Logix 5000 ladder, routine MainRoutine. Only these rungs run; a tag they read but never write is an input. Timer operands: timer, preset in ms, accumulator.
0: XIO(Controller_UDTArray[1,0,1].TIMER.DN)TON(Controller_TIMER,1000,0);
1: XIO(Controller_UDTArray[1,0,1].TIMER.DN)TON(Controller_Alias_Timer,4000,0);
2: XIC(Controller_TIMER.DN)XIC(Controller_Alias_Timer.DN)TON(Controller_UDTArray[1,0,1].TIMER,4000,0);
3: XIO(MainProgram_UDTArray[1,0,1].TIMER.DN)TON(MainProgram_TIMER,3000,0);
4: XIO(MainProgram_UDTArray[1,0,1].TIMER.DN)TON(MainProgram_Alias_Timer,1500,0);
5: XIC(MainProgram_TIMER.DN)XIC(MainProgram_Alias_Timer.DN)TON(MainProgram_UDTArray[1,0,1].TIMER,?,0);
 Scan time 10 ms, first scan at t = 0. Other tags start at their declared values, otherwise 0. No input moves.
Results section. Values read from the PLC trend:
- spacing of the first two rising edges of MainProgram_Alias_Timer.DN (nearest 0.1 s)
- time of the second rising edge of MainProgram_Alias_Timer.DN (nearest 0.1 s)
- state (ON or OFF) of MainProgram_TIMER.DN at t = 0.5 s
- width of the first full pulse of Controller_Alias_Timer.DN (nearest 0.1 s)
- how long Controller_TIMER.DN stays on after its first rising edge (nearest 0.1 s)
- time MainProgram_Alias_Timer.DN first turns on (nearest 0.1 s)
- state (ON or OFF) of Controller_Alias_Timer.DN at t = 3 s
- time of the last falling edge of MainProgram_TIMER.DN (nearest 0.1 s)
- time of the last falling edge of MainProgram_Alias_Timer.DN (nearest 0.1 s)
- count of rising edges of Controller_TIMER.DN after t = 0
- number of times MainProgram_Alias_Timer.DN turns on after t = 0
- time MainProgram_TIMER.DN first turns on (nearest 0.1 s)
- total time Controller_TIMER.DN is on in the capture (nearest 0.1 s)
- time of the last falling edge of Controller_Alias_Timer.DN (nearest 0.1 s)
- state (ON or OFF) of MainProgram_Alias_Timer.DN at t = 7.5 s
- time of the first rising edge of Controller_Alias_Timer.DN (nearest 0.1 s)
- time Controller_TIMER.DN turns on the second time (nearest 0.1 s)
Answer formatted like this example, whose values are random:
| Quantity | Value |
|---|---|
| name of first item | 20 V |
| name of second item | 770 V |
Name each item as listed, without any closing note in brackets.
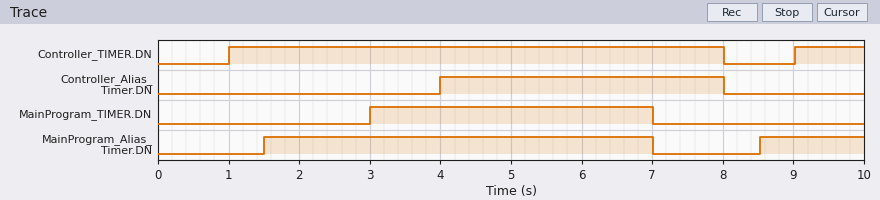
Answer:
| Quantity | Value |
|---|---|
| spacing of the first two rising edges of MainProgram_Alias_Timer.DN | 7.0 s |
| time of the second rising edge of MainProgram_Alias_Timer.DN | 8.5 s |
| state (ON or OFF) of MainProgram_TIMER.DN at t = 0.5 s | OFF |
| width of the first full pulse of Controller_Alias_Timer.DN | 4.0 s |
| how long Controller_TIMER.DN stays on after its first rising edge | 7.0 s |
| time MainProgram_Alias_Timer.DN first turns on | 1.5 s |
| state (ON or OFF) of Controller_Alias_Timer.DN at t = 3 s | OFF |
| time of the last falling edge of MainProgram_TIMER.DN | 7.0 s |
| time of the last falling edge of MainProgram_Alias_Timer.DN | 7.0 s |
| count of rising edges of Controller_TIMER.DN after t = 0 | 2 |
| number of times MainProgram_Alias_Timer.DN turns on after t = 0 | 2 |
| time MainProgram_TIMER.DN first turns on | 3.0 s |
| total time Controller_TIMER.DN is on in the capture | 8.0 s |
| time of the last falling edge of Controller_Alias_Timer.DN | 8.0 s |
| state (ON or OFF) of MainProgram_Alias_Timer.DN at t = 7.5 s | OFF |
| time of the first rising edge of Controller_Alias_Timer.DN | 4.0 s |
| time Controller_TIMER.DN turns on the second time | 9.0 s |
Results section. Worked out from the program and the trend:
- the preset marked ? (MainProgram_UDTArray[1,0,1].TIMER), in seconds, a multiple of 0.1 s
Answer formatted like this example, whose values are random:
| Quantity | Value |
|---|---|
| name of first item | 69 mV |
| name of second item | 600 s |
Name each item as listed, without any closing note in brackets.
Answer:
| Quantity | Value |
|---|---|
| the preset marked ? (MainProgram_UDTArray[1,0,1].TIMER), in seconds, a multiple of 0.1 s | 4.0 s |
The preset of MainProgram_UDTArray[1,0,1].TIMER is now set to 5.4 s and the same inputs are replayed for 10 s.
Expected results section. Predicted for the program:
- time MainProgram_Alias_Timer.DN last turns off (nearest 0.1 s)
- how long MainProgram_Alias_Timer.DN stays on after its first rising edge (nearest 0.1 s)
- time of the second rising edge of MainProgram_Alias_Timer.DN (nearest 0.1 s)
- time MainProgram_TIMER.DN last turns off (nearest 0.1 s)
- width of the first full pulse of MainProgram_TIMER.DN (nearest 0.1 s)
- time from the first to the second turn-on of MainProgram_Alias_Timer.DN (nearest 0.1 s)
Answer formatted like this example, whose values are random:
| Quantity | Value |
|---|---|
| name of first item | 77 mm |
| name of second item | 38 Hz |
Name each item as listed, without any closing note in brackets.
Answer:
| Quantity | Value |
|---|---|
| time MainProgram_Alias_Timer.DN last turns off | 8.4 s |
| how long MainProgram_Alias_Timer.DN stays on after its first rising edge | 6.9 s |
| time of the second rising edge of MainProgram_Alias_Timer.DN | 9.9 s |
| time MainProgram_TIMER.DN last turns off | 8.4 s |
| width of the first full pulse of MainProgram_TIMER.DN | 5.4 s |
| time from the first to the second turn-on of MainProgram_Alias_Timer.DN | 8.4 s |
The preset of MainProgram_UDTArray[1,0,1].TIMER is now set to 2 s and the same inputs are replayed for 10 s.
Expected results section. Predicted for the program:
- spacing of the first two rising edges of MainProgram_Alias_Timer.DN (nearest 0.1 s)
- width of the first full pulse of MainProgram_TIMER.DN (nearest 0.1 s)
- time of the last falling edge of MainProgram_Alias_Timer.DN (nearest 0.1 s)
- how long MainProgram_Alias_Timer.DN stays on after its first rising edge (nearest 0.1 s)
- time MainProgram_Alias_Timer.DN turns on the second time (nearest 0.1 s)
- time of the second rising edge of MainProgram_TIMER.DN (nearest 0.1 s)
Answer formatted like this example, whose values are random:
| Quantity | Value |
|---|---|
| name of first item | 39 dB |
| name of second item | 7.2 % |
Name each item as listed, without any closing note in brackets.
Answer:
| Quantity | Value |
|---|---|
| spacing of the first two rising edges of MainProgram_Alias_Timer.DN | 5.0 s |
| width of the first full pulse of MainProgram_TIMER.DN | 2.0 s |
| time of the last falling edge of MainProgram_Alias_Timer.DN | 5.0 s |
| how long MainProgram_Alias_Timer.DN stays on after its first rising edge | 3.5 s |
| time MainProgram_Alias_Timer.DN turns on the second time | 6.5 s |
| time of the second rising edge of MainProgram_TIMER.DN | 8.0 s |
